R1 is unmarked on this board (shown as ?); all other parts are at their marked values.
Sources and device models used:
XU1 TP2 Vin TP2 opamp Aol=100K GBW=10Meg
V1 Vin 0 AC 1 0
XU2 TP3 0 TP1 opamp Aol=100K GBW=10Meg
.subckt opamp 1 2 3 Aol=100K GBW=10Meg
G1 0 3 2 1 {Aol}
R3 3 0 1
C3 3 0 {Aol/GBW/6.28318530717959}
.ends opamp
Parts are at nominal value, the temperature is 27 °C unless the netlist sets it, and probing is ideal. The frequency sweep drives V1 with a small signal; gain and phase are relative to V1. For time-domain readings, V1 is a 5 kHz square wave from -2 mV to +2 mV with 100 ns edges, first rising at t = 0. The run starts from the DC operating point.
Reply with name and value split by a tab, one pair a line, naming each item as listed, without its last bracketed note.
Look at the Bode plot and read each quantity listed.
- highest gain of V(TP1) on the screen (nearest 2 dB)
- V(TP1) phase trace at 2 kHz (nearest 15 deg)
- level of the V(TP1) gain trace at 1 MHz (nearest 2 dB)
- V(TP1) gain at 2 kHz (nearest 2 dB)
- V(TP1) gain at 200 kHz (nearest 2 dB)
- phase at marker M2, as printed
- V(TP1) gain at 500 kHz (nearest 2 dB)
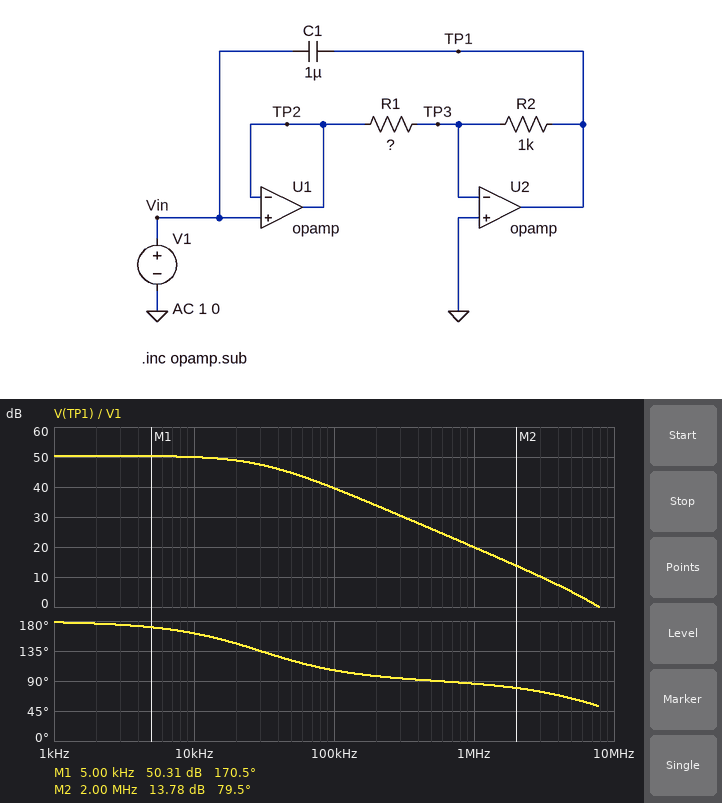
highest gain of V(TP1) on the screen	50 dB
V(TP1) phase trace at 2 kHz	180 deg
level of the V(TP1) gain trace at 1 MHz	20 dB
V(TP1) gain at 2 kHz	50 dB
V(TP1) gain at 200 kHz	34 dB
phase at marker M2, as printed	79.5 deg
V(TP1) gain at 500 kHz	26 dB
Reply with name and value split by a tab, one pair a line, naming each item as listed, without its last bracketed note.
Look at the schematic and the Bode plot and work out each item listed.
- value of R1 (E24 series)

value of R1	3 Ω
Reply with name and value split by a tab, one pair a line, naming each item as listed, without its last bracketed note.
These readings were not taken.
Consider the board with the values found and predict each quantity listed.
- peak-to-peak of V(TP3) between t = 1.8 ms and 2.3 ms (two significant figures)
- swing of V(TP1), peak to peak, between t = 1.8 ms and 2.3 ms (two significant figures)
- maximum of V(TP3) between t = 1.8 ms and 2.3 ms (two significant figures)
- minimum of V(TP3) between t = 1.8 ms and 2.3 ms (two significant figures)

peak-to-peak of V(TP3) between t = 1.8 ms and 2.3 ms	7.8 mV
swing of V(TP1), peak to peak, between t = 1.8 ms and 2.3 ms	1.3 V
maximum of V(TP3) between t = 1.8 ms and 2.3 ms	3.9 mV
minimum of V(TP3) between t = 1.8 ms and 2.3 ms	-3.9 mV
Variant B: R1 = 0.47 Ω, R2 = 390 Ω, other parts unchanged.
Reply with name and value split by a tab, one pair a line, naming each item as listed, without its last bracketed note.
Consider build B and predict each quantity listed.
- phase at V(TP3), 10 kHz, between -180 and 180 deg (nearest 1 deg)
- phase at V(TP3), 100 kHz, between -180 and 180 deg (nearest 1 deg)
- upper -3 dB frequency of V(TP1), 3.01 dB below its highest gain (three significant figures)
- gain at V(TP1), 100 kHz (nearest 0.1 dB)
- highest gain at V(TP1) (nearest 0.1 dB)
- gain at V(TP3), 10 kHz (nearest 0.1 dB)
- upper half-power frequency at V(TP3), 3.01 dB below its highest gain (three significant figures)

phase at V(TP3), 10 kHz, between -180 and 180 deg	50 deg
phase at V(TP3), 100 kHz, between -180 and 180 deg	6 deg
upper -3 dB frequency of V(TP1), 3.01 dB below its highest gain	12.1 kHz
gain at V(TP1), 100 kHz	39.9 dB
highest gain at V(TP1)	58.3 dB
gain at V(TP3), 10 kHz	-3.9 dB
upper half-power frequency at V(TP3), 3.01 dB below its highest gain	10.0 MHz
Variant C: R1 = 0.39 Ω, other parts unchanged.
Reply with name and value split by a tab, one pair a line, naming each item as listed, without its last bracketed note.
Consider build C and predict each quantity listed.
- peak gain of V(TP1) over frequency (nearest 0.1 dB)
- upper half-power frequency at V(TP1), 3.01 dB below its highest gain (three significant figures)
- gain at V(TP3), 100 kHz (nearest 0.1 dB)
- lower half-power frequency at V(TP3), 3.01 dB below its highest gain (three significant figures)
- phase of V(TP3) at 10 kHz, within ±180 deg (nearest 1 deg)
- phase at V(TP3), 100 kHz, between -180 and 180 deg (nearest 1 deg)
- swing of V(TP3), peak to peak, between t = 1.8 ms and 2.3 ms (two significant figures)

peak gain of V(TP1) over frequency	68.0 dB
upper half-power frequency at V(TP1), 3.01 dB below its highest gain	4.00 kHz
gain at V(TP3), 100 kHz	0 dB
lower half-power frequency at V(TP3), 3.01 dB below its highest gain	3.99 kHz
phase of V(TP3) at 10 kHz, within ±180 deg	21 deg
phase at V(TP3), 100 kHz, between -180 and 180 deg	2 deg
swing of V(TP3), peak to peak, between t = 1.8 ms and 2.3 ms	7.3 mV
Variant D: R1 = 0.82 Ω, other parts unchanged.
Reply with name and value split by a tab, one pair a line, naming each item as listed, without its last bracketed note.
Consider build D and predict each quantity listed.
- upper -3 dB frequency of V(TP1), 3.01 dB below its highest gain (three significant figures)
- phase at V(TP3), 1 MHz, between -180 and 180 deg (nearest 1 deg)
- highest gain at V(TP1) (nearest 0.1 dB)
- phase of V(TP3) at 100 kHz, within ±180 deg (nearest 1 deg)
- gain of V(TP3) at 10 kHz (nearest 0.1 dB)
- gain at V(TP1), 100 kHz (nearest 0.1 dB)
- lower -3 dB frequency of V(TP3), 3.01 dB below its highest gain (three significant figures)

upper -3 dB frequency of V(TP1), 3.01 dB below its highest gain	8.29 kHz
phase at V(TP3), 1 MHz, between -180 and 180 deg	-5 deg
highest gain at V(TP1)	61.6 dB
phase of V(TP3) at 100 kHz, within ±180 deg	4 deg
gain of V(TP3) at 10 kHz	-2.3 dB
gain at V(TP1), 100 kHz	40.0 dB
lower -3 dB frequency of V(TP3), 3.01 dB below its highest gain	8.27 kHz
